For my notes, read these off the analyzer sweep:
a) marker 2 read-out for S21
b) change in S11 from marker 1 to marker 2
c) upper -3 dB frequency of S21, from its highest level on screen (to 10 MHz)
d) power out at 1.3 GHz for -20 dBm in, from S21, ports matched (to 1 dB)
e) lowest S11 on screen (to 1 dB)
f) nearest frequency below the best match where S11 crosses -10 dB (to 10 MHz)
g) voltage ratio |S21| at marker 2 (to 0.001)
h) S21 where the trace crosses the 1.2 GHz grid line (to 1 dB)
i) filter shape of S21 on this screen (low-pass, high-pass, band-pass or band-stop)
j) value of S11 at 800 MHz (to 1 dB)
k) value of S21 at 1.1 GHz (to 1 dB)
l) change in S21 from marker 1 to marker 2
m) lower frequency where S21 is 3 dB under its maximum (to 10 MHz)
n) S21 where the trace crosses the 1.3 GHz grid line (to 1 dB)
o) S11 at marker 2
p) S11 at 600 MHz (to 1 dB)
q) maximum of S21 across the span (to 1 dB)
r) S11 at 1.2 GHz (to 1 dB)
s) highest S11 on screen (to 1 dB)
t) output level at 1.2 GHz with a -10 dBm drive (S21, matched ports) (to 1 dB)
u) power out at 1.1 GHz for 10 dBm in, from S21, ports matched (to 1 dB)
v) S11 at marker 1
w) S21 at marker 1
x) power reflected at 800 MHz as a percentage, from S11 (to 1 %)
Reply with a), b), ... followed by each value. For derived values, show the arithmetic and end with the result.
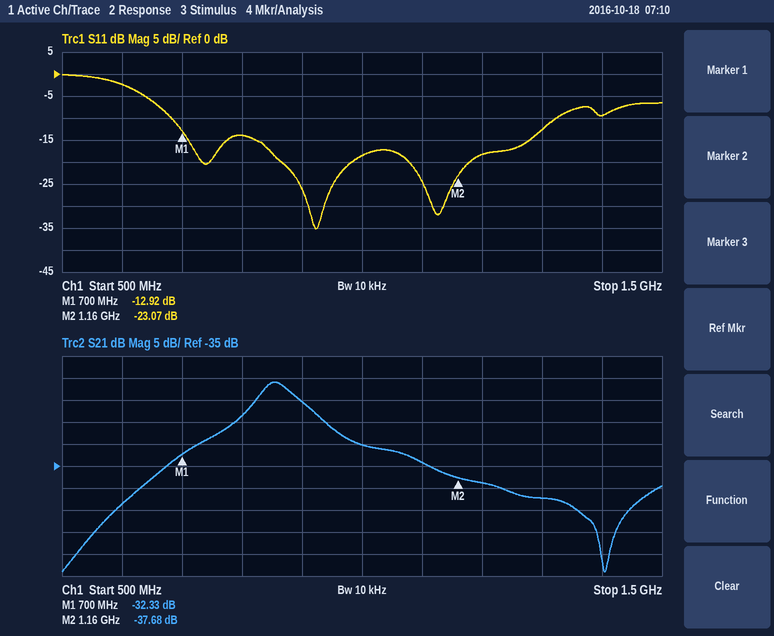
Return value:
a) -37.68 dB
b) -23.07 − (-12.92) = -10.15 dB
c) 890 MHz
d) -20 dBm + (-42 dB) = -62 dBm
e) -35 dB
f) 680 MHz
g) 10^(-37.68/20) ≈ 0.013
h) -39 dB
i) band-pass
j) -14 dB
k) -34 dB
l) -37.68 − (-32.33) = -5.35 dB
m) 830 MHz
n) -42 dB
o) -23.07 dB
p) -2 dB
q) -16 dB
r) -18 dB
s) 0 dB
t) -10 dBm + (-39 dB) = -49 dBm
u) 10 dBm + (-34 dB) = -24 dBm
v) -12.92 dB
w) -32.33 dB
x) 10^(-14/10) ≈ 4 %
